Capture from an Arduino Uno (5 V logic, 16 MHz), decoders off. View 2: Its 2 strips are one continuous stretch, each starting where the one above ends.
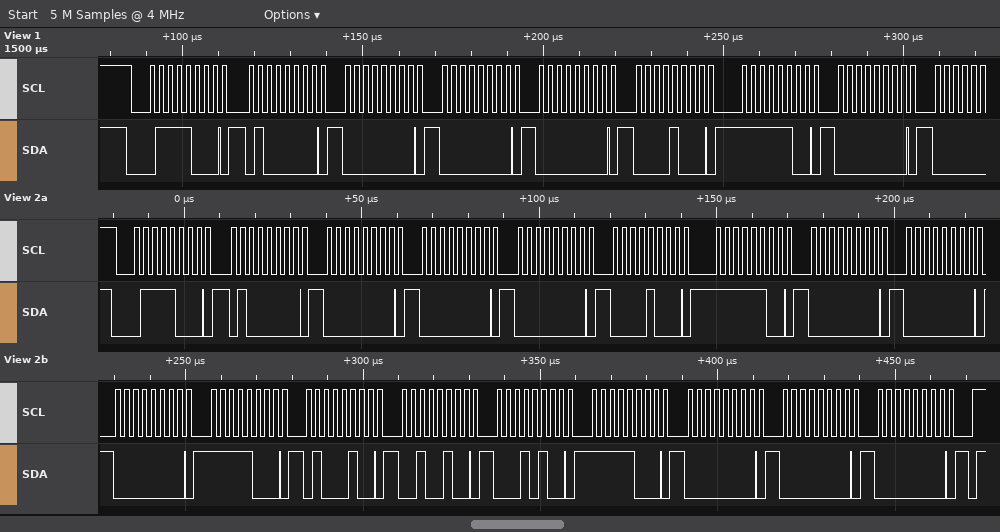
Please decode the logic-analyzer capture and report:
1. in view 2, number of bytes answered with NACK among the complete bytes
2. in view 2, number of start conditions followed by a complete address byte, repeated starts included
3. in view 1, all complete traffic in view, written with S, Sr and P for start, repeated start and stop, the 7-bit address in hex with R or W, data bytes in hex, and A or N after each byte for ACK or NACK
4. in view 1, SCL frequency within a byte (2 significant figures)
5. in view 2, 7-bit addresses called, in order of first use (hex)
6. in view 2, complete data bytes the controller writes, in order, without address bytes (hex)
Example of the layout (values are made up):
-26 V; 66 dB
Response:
0; 1; S 3CW A 40 A 00 A 00 A 00 A 08 A FC A 00 A; 400 kHz; 0x3C; 40 00 00 00 08 FC 00 00 00 F8 44 24 14 F8 00 00 00
